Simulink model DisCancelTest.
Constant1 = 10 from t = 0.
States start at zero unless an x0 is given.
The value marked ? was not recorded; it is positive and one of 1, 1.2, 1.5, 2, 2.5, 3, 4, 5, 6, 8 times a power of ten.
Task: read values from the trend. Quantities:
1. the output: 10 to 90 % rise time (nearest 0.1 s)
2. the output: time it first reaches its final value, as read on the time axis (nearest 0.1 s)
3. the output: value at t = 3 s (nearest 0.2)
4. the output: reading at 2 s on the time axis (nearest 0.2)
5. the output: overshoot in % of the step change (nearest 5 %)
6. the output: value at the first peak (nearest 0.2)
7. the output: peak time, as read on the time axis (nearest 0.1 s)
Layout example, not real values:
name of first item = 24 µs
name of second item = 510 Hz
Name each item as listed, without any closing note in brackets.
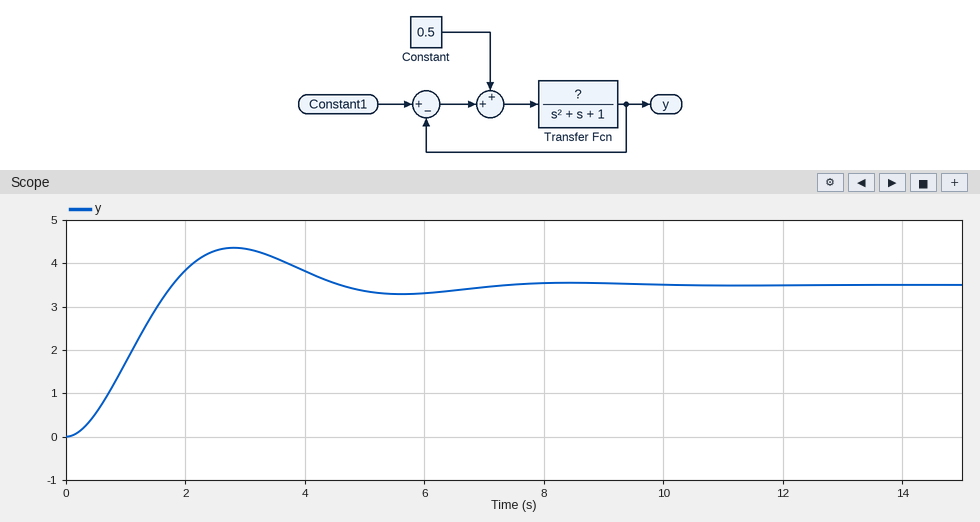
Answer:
the output: 10 to 90 % rise time = 1.2 s
the output: time it first reaches its final value, as read on the time axis = 1.8 s
the output: value at t = 3 s = 4.4
the output: reading at 2 s on the time axis = 3.8
the output: overshoot in % of the step change = 25 %
the output: value at the first peak = 4.4
the output: peak time, as read on the time axis = 2.8 s
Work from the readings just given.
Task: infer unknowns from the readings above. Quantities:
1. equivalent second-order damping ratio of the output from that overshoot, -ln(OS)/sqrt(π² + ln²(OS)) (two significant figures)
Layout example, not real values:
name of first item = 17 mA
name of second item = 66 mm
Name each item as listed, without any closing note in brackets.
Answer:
equivalent second-order damping ratio of the output from that overshoot, -ln(OS)/sqrt(π² + ln²(OS)) = 0.40
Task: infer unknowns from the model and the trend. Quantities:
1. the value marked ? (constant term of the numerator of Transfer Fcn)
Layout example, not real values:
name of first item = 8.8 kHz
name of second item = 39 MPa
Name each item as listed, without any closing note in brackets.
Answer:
the value marked ? = 0.5
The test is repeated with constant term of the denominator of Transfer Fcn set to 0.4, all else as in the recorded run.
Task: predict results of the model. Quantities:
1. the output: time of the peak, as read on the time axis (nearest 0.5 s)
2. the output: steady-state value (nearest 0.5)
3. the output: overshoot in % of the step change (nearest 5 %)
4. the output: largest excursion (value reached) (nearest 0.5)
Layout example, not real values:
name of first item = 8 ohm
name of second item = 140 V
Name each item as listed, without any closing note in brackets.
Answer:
the output: time of the peak, as read on the time axis = 4.0 s
the output: steady-state value = 6.0
the output: overshoot in % of the step change = 15 %
the output: largest excursion (value reached) = 6.5
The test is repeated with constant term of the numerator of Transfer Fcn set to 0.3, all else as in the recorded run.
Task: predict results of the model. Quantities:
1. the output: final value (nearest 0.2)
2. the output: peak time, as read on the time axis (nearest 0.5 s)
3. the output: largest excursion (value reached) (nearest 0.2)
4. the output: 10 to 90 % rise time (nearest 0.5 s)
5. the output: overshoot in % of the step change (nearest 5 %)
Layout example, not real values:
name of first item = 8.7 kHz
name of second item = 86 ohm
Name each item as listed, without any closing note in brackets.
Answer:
the output: final value = 2.4
the output: peak time, as read on the time axis = 3.0 s
the output: largest excursion (value reached) = 3.0
the output: 10 to 90 % rise time = 1.5 s
the output: overshoot in % of the step change = 20 %
